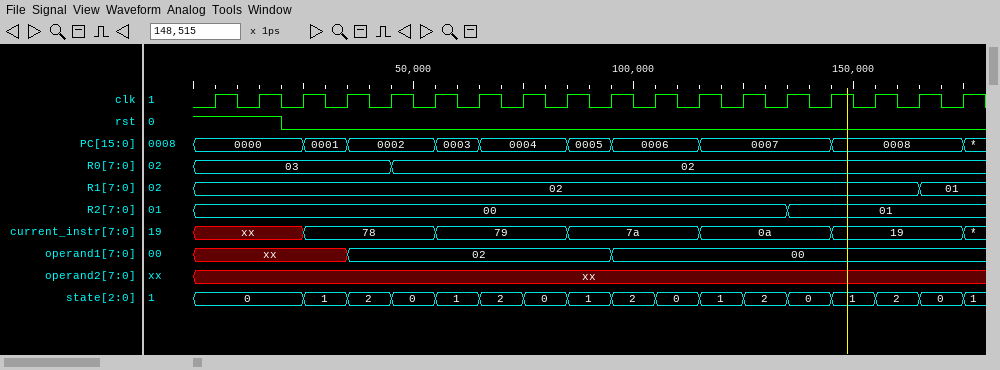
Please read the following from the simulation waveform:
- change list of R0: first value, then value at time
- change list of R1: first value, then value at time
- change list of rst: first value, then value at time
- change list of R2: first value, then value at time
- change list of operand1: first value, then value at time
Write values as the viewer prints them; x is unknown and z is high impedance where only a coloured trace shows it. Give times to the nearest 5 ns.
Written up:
03, 02 at 45 ns
02, 01 at 165 ns
1, 0 at 20 ns
00, 01 at 135 ns
xx, 02 at 35 ns, 00 at 95 ns
